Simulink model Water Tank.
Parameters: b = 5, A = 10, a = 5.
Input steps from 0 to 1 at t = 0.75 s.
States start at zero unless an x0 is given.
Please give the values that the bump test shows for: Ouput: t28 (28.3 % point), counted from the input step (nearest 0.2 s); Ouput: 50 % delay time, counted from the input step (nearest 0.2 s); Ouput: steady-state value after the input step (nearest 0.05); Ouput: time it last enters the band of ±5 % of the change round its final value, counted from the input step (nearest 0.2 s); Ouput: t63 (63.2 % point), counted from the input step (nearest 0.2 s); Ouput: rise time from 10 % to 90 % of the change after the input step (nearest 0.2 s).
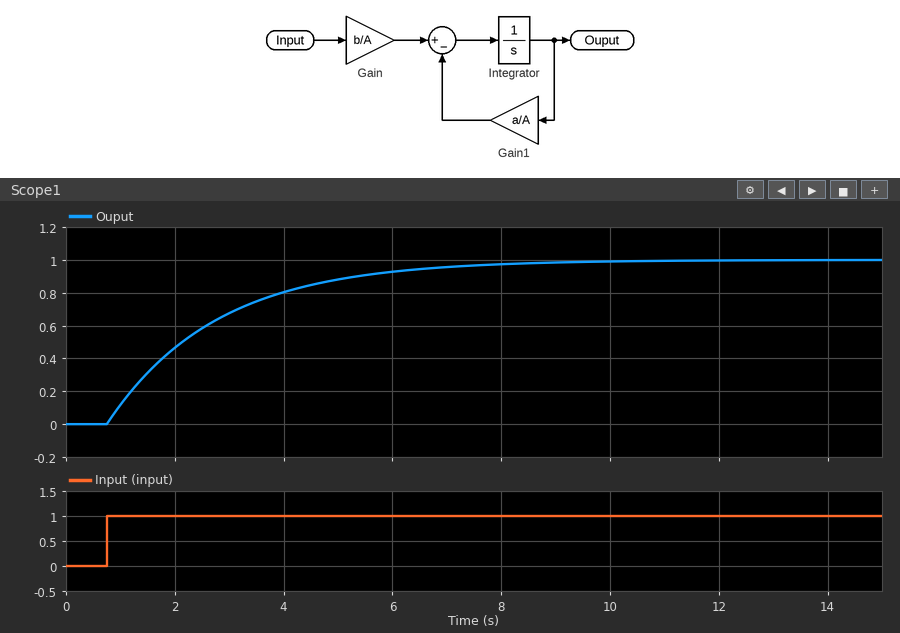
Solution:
0.6 s
1.4 s
1.00
6.0 s
2.0 s
4.4 s
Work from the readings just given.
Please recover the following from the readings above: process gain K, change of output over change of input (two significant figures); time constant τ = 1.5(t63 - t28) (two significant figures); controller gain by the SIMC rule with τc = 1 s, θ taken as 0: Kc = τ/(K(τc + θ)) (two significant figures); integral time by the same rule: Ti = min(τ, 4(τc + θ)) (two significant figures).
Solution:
1.0
2.1 s
2.1
2.1 s
